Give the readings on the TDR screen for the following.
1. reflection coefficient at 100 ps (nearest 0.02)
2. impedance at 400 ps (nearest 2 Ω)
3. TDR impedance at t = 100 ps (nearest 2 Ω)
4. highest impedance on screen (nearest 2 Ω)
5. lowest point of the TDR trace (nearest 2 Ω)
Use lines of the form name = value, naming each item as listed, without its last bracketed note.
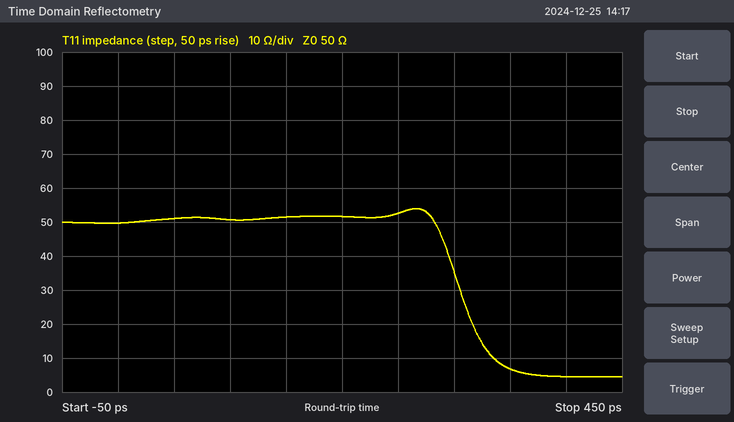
reflection coefficient at 100 ps = 0.00
impedance at 400 ps = 4 Ω
TDR impedance at t = 100 ps = 50 Ω
highest impedance on screen = 54 Ω
lowest point of the TDR trace = 4 Ω
